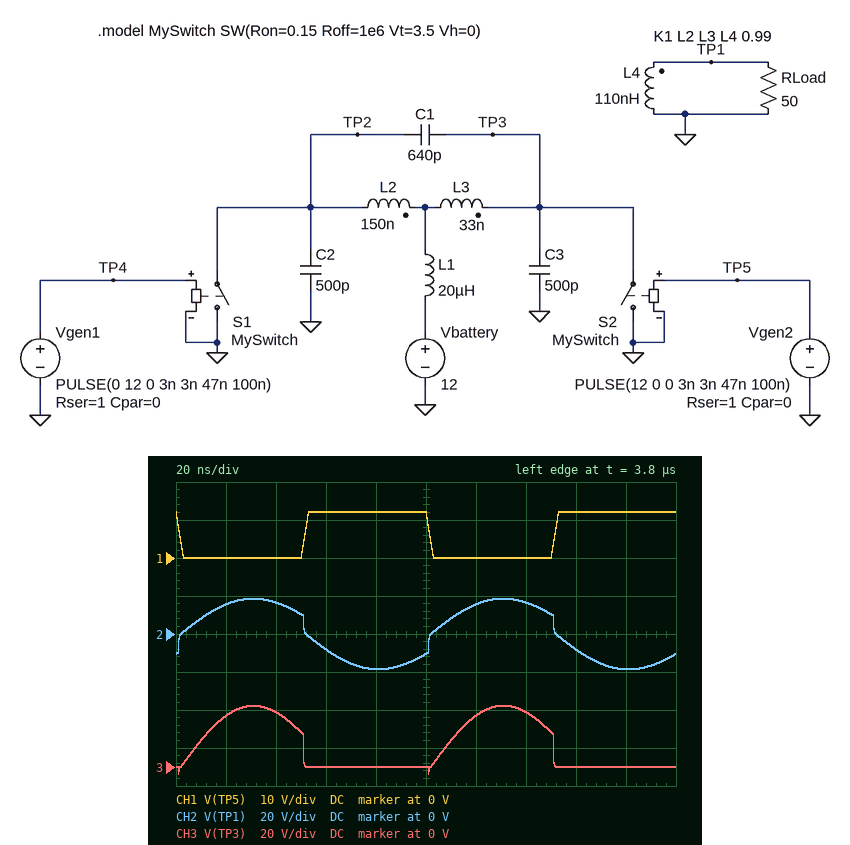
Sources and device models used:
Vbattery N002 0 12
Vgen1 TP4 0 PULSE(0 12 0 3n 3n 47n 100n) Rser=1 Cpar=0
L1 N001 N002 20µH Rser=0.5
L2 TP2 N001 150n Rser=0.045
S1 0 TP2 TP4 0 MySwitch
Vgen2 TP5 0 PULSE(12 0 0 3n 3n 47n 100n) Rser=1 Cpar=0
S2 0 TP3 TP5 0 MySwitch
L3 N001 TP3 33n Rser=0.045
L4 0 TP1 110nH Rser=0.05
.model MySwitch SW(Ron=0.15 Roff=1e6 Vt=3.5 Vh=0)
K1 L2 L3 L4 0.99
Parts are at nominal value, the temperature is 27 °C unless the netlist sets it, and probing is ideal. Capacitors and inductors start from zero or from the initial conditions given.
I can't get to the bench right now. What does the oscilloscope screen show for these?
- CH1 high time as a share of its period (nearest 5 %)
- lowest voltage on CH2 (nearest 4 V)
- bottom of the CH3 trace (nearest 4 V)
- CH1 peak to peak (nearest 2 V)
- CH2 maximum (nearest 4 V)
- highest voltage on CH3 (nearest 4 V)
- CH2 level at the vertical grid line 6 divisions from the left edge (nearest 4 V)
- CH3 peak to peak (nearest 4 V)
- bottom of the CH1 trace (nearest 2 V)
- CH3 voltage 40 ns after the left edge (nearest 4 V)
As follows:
50 %
-20 V
-4 V
12 V
20 V
32 V
16 V
36 V
0 V
28 V
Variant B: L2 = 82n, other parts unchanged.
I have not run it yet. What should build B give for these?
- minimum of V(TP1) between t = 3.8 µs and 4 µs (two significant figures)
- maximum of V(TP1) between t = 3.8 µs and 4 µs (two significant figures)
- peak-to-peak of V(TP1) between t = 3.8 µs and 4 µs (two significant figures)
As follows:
-26 V
26 V
51 V
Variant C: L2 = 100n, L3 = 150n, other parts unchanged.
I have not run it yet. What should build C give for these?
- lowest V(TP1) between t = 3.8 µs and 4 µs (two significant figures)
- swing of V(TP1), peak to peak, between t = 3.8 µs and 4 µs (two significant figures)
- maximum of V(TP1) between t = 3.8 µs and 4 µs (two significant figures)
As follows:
-14 V
27 V
14 V
